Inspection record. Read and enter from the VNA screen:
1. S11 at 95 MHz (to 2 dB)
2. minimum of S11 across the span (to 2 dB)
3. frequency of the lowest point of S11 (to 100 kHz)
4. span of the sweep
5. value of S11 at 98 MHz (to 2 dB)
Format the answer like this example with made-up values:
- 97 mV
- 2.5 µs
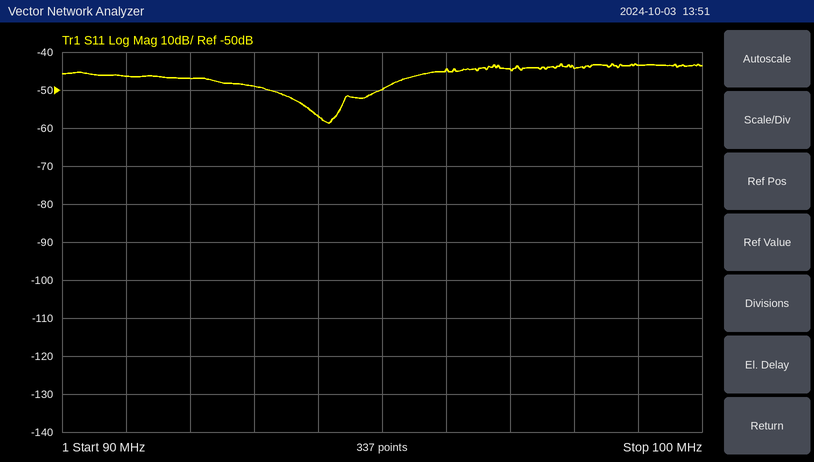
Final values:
- -50 dB
- -58 dB
- 94.2 MHz
- 10 MHz
- -44 dB
